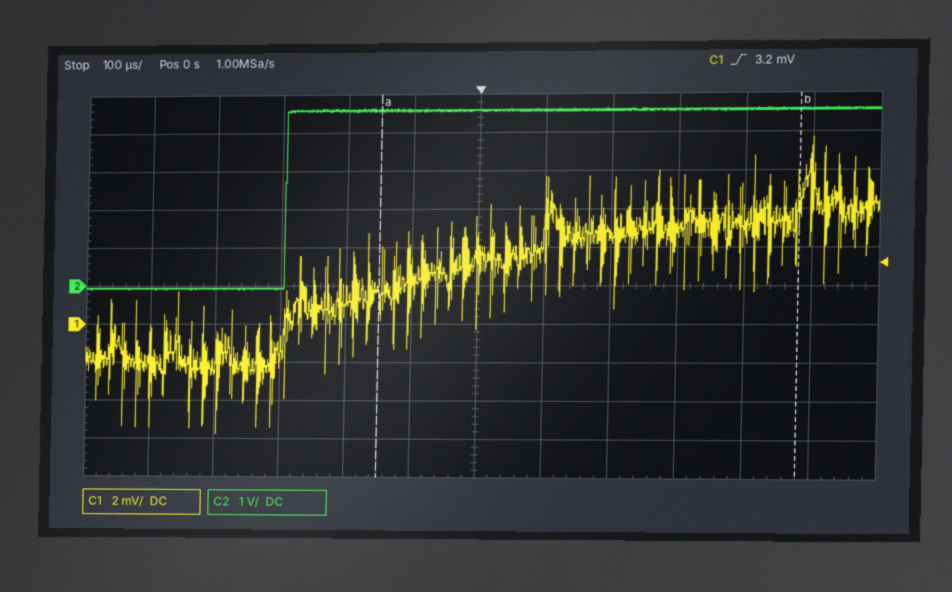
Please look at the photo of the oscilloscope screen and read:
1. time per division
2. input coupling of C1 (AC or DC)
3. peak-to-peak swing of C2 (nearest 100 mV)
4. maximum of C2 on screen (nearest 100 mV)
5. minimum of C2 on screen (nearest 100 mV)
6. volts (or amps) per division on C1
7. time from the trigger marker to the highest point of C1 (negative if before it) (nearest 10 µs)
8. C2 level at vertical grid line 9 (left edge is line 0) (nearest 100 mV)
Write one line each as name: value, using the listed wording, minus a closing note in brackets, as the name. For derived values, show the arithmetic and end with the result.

time per division: 100 µs
input coupling of C1: DC
peak-to-peak swing of C2: 4.6 V − (-100 mV) = 4.7 V
maximum of C2 on screen: 4.6 V
minimum of C2 on screen: -100 mV
volts (or amps) per division on C1: 2 mV
time from the trigger marker to the highest point of C1 (negative if before it): +500 µs
C2 level at vertical grid line 9 (left edge is line 0): 4.6 V
